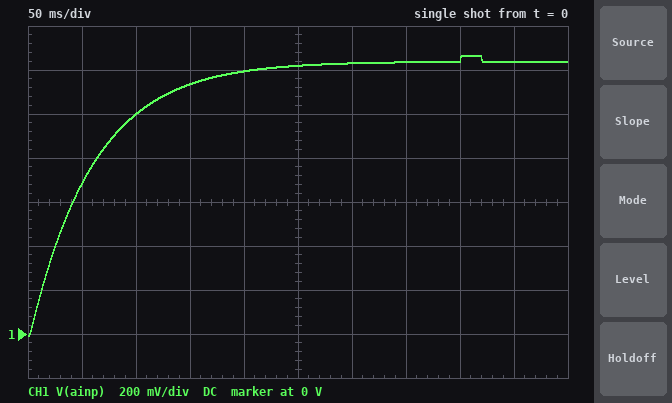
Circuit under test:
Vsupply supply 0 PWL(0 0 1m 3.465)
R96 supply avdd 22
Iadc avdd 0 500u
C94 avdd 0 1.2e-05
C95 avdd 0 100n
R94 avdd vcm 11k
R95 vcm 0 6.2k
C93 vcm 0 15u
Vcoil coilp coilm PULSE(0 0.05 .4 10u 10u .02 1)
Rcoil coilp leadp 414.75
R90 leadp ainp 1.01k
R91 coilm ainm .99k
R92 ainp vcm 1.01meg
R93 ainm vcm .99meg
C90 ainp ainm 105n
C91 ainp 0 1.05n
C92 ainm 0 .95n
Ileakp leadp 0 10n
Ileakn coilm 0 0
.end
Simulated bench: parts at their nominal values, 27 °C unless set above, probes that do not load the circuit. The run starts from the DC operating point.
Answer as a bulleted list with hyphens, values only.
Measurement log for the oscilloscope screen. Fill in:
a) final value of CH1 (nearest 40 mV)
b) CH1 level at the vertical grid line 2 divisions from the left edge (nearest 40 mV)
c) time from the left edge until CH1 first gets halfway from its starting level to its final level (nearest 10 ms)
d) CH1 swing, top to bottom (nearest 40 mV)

- 1.24 V
- 1.00 V
- 40 ms
- 1.28 V
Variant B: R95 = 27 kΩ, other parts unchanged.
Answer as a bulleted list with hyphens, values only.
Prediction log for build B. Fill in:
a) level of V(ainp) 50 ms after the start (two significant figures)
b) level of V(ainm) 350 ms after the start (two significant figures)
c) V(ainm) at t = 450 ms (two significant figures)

- 820 mV
- 2.3 V
- 2.4 V
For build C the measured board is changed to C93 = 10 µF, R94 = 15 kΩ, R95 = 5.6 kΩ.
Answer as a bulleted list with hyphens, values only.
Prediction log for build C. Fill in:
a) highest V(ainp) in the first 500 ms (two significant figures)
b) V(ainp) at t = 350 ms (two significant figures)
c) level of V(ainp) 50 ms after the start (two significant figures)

- 960 mV
- 930 mV
- 640 mV
